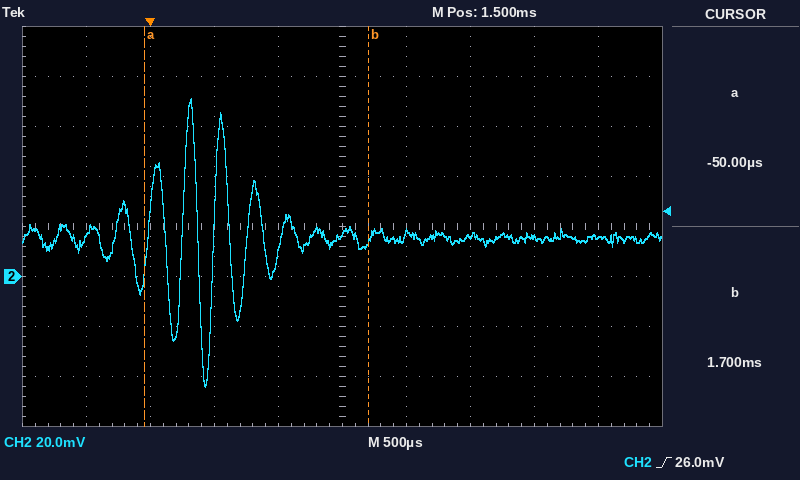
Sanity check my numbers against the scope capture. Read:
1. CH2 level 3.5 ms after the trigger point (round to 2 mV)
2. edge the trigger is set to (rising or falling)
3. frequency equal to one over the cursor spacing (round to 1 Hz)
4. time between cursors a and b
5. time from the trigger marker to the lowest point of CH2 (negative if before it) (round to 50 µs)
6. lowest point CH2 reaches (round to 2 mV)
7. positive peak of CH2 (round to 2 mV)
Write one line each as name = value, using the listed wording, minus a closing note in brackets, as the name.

CH2 level 3.5 ms after the trigger point = 16 mV
edge the trigger is set to = rising
frequency equal to one over the cursor spacing = 571 Hz
time between cursors a and b = 1.75 ms
time from the trigger marker to the lowest point of CH2 (negative if before it) = +450 µs
lowest point CH2 reaches = -44 mV
positive peak of CH2 = 72 mV
